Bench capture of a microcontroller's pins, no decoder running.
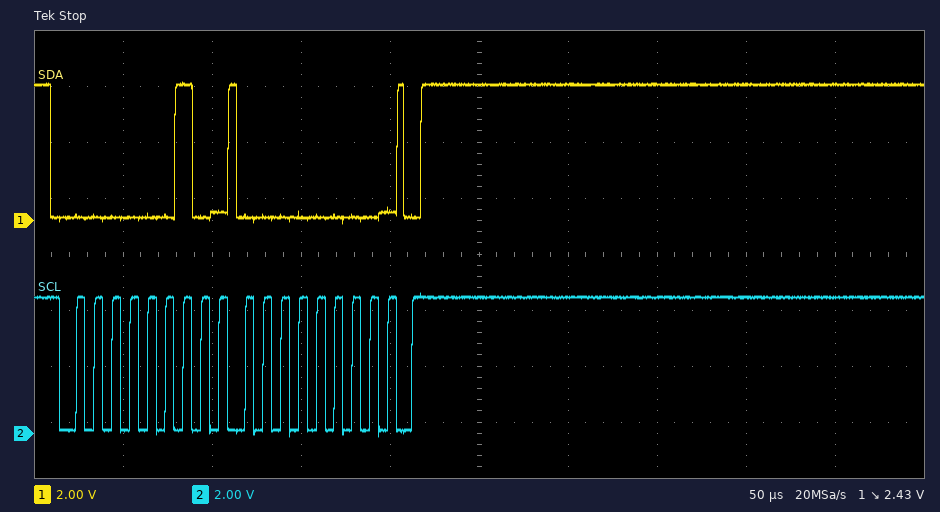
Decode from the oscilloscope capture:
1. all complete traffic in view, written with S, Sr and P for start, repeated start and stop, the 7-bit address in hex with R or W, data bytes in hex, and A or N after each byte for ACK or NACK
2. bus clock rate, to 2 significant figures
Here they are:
S 01W A 00 A P
100 kHz
